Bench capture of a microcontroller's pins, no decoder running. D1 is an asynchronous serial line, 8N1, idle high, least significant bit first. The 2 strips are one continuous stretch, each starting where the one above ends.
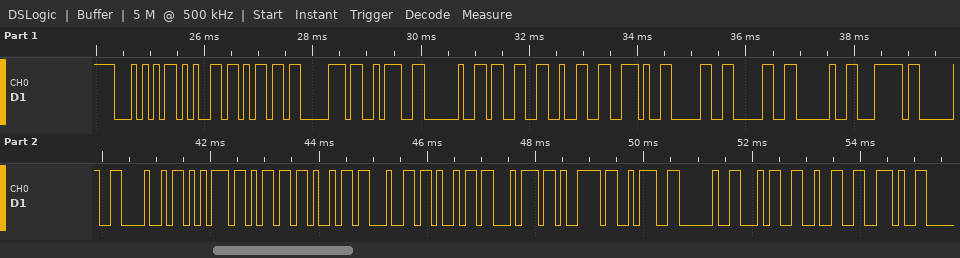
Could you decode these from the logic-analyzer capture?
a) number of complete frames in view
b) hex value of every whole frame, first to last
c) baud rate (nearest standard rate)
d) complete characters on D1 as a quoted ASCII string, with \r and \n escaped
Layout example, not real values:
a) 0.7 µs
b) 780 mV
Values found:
a) 27
b) 54 65 6D 70 3A 20 33 32 2E 30 30 20 7C 20 48 75 6D 69 64 69 74 79 3A 20 34 32 2E
c) 9600 baud
d) "Temp: 32.00 | Humidity: 42."
